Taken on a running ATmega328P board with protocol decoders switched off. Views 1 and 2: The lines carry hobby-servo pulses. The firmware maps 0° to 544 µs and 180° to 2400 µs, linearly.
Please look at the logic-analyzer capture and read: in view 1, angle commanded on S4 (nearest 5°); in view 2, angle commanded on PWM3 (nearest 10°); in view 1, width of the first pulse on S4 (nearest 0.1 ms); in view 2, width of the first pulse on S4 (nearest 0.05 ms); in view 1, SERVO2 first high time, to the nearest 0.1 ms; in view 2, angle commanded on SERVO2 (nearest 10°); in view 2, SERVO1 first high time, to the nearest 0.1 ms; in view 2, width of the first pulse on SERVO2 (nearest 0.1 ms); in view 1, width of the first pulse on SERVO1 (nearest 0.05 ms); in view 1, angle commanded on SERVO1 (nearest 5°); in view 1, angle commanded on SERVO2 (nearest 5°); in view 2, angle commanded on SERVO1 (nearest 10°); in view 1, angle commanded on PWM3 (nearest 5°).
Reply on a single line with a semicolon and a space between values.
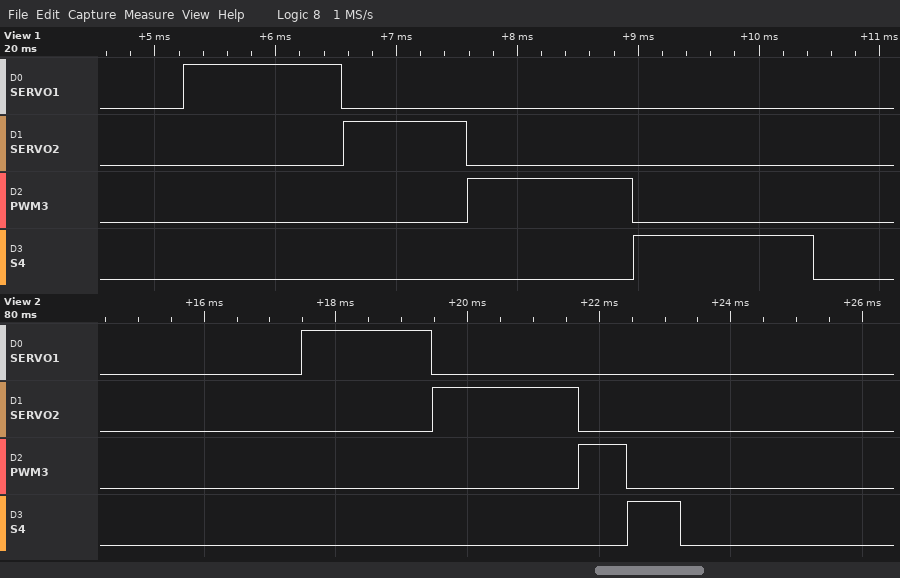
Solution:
90°; 20°; 1.5 ms; 0.80 ms; 1.0 ms; 160°; 2.0 ms; 2.2 ms; 1.30 ms; 75°; 45°; 140°; 80°
